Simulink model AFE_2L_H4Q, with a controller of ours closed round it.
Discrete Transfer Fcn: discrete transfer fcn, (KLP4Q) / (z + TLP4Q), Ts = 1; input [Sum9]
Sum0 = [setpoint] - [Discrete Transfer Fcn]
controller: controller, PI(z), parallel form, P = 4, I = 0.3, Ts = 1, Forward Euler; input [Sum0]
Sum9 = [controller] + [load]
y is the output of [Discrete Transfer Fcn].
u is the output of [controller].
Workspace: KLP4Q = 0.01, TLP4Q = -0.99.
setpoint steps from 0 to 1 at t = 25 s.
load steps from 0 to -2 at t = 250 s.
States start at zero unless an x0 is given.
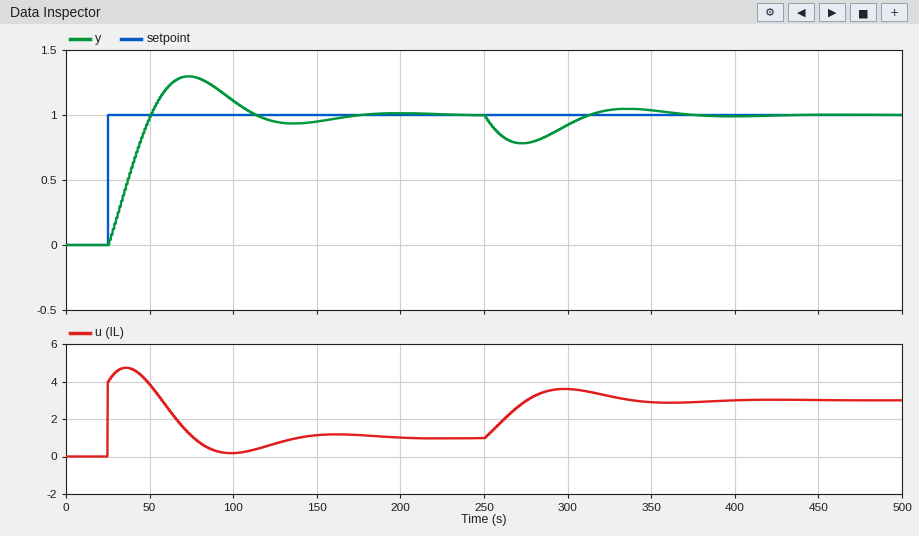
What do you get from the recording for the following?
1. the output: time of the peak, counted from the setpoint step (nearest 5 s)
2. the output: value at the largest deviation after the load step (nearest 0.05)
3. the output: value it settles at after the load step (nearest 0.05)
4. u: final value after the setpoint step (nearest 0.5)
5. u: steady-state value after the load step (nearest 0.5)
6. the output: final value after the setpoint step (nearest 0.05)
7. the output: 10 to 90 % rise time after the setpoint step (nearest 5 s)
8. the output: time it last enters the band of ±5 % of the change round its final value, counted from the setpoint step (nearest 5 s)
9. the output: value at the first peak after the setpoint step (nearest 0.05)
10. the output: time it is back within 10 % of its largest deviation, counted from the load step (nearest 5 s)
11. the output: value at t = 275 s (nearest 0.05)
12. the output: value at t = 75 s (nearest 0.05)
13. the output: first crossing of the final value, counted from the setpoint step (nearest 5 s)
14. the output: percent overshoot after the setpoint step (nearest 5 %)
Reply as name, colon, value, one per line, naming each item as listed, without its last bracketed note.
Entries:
the output: time of the peak, counted from the setpoint step: 50 s
the output: value at the largest deviation after the load step: 0.80
the output: value it settles at after the load step: 1.00
u: final value after the setpoint step: 1.0
u: steady-state value after the load step: 3.0
the output: final value after the setpoint step: 1.00
the output: 10 to 90 % rise time after the setpoint step: 20 s
the output: time it last enters the band of ±5 % of the change round its final value, counted from the setpoint step: 125 s
the output: value at the first peak after the setpoint step: 1.30
the output: time it is back within 10 % of its largest deviation, counted from the load step: 110 s
the output: value at t = 275 s: 0.80
the output: value at t = 75 s: 1.30
the output: first crossing of the final value, counted from the setpoint step: 25 s
the output: percent overshoot after the setpoint step: 30 %
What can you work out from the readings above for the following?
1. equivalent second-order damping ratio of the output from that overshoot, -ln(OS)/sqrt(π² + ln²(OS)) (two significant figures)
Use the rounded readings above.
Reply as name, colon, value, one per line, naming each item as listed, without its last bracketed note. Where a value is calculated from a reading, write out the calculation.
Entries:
equivalent second-order damping ratio of the output from that overshoot, -ln(OS)/sqrt(π² + ln²(OS)): ln(0.3) = -1.204; 1.204 / sqrt(9.870 + 1.450) = 0.36
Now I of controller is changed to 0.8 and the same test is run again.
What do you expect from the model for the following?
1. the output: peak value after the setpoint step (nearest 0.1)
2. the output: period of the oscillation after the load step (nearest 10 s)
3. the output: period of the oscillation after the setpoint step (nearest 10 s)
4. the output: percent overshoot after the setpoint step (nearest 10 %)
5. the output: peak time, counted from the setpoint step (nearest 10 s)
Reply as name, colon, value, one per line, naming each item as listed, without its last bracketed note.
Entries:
the output: peak value after the setpoint step: 1.5
the output: period of the oscillation after the load step: 70 s
the output: period of the oscillation after the setpoint step: 70 s
the output: percent overshoot after the setpoint step: 50 %
the output: peak time, counted from the setpoint step: 30 s
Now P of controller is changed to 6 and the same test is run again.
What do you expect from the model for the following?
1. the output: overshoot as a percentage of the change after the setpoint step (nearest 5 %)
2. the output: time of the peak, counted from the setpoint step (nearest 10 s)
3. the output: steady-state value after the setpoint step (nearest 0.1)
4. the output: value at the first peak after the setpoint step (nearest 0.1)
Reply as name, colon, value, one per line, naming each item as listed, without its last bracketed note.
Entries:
the output: overshoot as a percentage of the change after the setpoint step: 20 %
the output: time of the peak, counted from the setpoint step: 40 s
the output: steady-state value after the setpoint step: 1.0
the output: value at the first peak after the setpoint step: 1.2
